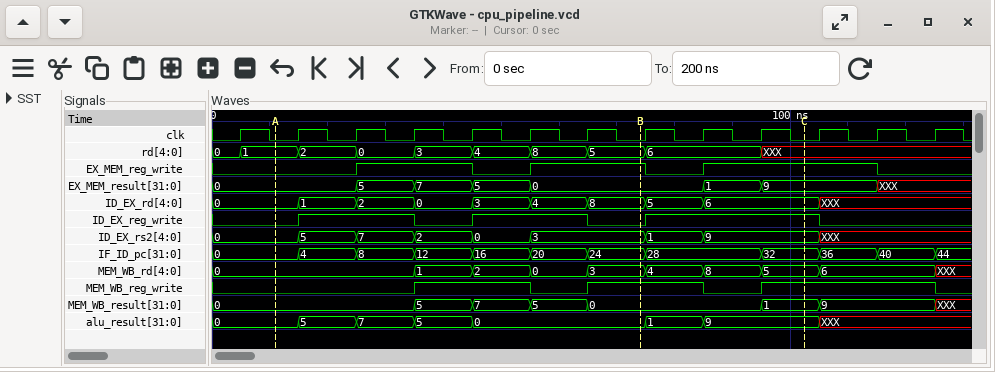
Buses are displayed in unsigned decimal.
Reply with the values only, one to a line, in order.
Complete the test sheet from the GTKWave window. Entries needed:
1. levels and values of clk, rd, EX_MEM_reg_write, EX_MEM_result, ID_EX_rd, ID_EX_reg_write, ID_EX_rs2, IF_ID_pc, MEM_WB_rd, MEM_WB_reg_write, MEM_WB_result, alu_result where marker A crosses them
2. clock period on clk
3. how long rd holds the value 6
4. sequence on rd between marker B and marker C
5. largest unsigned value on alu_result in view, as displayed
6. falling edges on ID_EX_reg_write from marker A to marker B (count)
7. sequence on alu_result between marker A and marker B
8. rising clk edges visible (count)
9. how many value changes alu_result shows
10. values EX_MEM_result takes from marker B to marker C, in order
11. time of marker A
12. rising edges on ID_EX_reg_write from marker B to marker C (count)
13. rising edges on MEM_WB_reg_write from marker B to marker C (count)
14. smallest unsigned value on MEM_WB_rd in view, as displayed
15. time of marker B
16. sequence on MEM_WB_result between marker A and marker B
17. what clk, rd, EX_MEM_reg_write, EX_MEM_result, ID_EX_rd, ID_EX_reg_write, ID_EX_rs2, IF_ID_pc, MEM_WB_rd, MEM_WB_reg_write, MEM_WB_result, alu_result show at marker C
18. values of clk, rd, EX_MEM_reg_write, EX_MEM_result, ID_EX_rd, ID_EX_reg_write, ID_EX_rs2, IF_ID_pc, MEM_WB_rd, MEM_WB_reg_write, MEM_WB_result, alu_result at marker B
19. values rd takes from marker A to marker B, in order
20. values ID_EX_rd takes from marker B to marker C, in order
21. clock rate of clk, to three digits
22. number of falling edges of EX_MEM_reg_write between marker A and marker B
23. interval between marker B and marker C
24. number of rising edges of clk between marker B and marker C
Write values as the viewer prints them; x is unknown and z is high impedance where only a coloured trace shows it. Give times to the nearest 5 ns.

clk=0, rd=1, EX_MEM_reg_write=0, EX_MEM_result=0, ID_EX_rd=0, ID_EX_reg_write=0, ID_EX_rs2=0, IF_ID_pc=0, MEM_WB_rd=0, MEM_WB_reg_write=0, MEM_WB_result=0, alu_result=0
10 ns
20 ns
5, 6, XXX
9
2
0, 5, 7, 5, 0
13
7
0, 1, 9
10 ns
1
1
0
75 ns
0, 5, 7, 5, 0
clk=0, rd=XXX, EX_MEM_reg_write=1, EX_MEM_result=9, ID_EX_rd=6, ID_EX_reg_write=1, ID_EX_rs2=9, IF_ID_pc=32, MEM_WB_rd=5, MEM_WB_reg_write=1, MEM_WB_result=1, alu_result=9
clk=0, rd=5, EX_MEM_reg_write=1, EX_MEM_result=0, ID_EX_rd=8, ID_EX_reg_write=0, ID_EX_rs2=3, IF_ID_pc=24, MEM_WB_rd=3, MEM_WB_reg_write=1, MEM_WB_result=0, alu_result=0
1, 2, 0, 3, 4, 8, 5
8, 5, 6
100 MHz
1
30 ns
3
